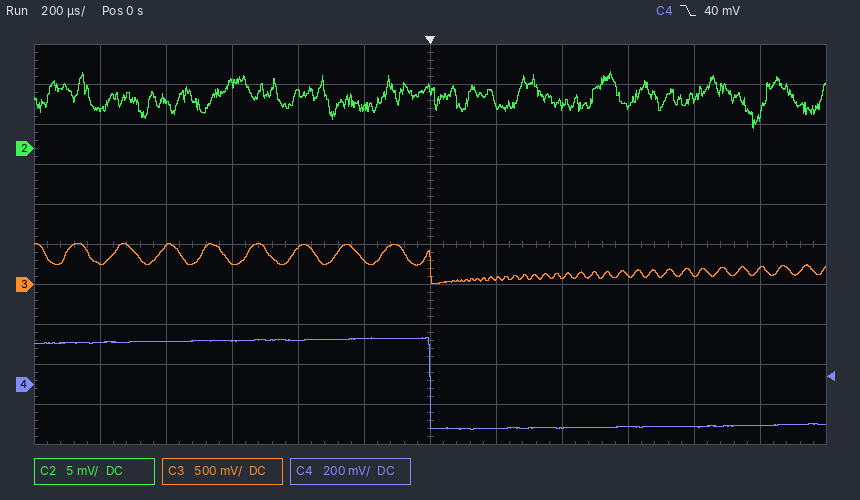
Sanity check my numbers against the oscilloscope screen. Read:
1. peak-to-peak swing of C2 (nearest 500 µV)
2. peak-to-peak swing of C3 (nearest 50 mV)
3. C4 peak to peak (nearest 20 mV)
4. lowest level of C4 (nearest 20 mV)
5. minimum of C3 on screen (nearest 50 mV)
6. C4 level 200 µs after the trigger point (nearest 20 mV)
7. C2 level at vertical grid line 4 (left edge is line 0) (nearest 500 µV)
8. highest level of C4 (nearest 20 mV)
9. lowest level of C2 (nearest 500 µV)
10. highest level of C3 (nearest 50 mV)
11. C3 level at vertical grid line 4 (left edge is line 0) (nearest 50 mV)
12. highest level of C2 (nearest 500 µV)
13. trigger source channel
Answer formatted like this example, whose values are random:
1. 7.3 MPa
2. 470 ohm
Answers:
1. 7.0 mV
2. 500 mV
3. 460 mV
4. -220 mV
5. 0 mV
6. -220 mV
7. 7.0 mV
8. 240 mV
9. 2.5 mV
10. 500 mV
11. 450 mV
12. 9.5 mV
13. C4
